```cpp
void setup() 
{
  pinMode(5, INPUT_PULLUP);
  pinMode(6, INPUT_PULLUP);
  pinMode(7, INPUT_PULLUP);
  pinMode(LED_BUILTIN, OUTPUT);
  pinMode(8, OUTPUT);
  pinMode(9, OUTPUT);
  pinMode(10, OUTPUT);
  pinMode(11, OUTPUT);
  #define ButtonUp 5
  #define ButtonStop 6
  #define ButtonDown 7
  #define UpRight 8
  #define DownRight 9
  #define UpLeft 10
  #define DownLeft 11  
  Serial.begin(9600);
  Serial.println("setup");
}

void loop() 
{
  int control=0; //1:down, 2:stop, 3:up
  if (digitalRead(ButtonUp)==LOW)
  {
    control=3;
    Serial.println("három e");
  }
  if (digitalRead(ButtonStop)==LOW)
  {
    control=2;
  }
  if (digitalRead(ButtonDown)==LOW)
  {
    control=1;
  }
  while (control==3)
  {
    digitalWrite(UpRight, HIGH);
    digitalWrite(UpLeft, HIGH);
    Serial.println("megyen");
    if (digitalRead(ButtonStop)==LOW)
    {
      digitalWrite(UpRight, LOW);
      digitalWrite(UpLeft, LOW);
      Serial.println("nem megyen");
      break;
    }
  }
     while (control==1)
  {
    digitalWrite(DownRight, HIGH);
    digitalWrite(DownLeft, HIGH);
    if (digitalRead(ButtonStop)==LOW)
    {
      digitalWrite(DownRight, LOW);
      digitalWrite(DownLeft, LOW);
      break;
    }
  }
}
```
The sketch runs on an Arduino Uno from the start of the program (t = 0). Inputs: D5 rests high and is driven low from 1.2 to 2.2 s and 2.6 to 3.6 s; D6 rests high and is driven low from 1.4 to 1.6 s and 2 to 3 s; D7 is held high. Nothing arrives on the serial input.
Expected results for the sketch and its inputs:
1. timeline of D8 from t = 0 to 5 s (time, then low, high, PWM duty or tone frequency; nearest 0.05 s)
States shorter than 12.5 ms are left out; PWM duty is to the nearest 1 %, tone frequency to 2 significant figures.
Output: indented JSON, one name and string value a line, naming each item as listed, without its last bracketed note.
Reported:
{
  "timeline of D8 from t = 0 to 5 s": "0 s low; 1.2 s high; 1.4 s low; 1.6 s high; 2 s low; 3 s high"
}
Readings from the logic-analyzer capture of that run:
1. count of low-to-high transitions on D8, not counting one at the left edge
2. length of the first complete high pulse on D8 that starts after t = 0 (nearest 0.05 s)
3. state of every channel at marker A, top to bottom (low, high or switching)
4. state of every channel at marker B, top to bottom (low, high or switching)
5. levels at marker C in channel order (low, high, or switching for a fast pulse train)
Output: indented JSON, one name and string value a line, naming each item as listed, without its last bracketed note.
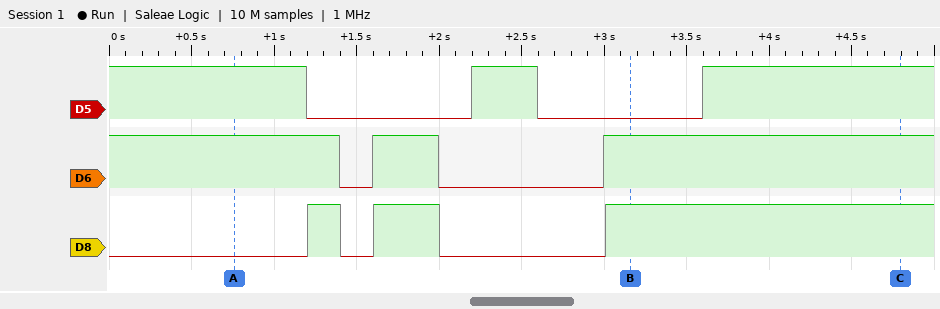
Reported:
{
  "count of low-to-high transitions on D8, not counting one at the left edge": "3",
  "length of the first complete high pulse on D8 that starts after t = 0": "0.20 s",
  "state of every channel at marker A, top to bottom": "D5 high, D6 high, D8 low",
  "state of every channel at marker B, top to bottom": "D5 low, D6 high, D8 high",
  "levels at marker C in channel order": "D5 high, D6 high, D8 high"
}
